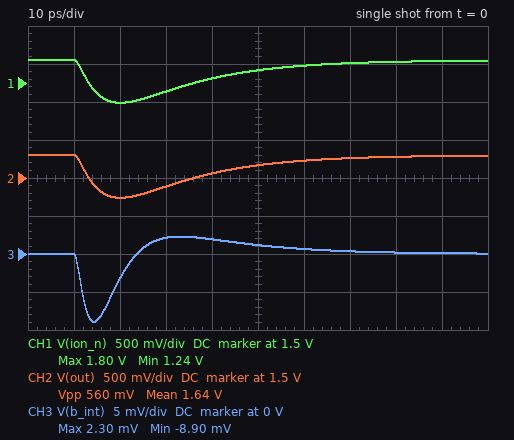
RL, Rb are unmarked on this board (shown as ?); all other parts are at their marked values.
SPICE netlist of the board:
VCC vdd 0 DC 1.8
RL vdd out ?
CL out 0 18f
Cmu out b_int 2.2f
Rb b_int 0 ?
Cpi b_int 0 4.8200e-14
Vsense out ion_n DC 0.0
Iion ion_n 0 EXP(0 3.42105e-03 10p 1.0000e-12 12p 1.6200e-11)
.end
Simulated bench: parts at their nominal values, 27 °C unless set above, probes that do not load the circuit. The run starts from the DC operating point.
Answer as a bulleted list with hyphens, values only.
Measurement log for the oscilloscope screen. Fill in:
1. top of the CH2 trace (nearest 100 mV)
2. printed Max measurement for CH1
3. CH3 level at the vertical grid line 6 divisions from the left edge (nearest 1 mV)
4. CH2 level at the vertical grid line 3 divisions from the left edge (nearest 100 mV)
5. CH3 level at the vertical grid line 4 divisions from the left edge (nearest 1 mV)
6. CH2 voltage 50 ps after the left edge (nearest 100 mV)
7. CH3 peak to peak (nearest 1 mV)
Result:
- 1.8 V
- 1.80 V
- 1 mV
- 1.4 V
- 2 mV
- 1.7 V
- 11 mV
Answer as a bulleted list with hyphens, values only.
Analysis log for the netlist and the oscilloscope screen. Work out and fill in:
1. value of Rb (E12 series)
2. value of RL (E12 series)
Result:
- 56 Ω
- 270 Ω
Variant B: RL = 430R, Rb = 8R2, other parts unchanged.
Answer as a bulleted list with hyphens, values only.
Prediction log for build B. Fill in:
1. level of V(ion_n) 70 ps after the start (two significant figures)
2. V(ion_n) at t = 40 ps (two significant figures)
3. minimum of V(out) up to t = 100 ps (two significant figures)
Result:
- 1.7 V
- 1.4 V
- 1.0 V
